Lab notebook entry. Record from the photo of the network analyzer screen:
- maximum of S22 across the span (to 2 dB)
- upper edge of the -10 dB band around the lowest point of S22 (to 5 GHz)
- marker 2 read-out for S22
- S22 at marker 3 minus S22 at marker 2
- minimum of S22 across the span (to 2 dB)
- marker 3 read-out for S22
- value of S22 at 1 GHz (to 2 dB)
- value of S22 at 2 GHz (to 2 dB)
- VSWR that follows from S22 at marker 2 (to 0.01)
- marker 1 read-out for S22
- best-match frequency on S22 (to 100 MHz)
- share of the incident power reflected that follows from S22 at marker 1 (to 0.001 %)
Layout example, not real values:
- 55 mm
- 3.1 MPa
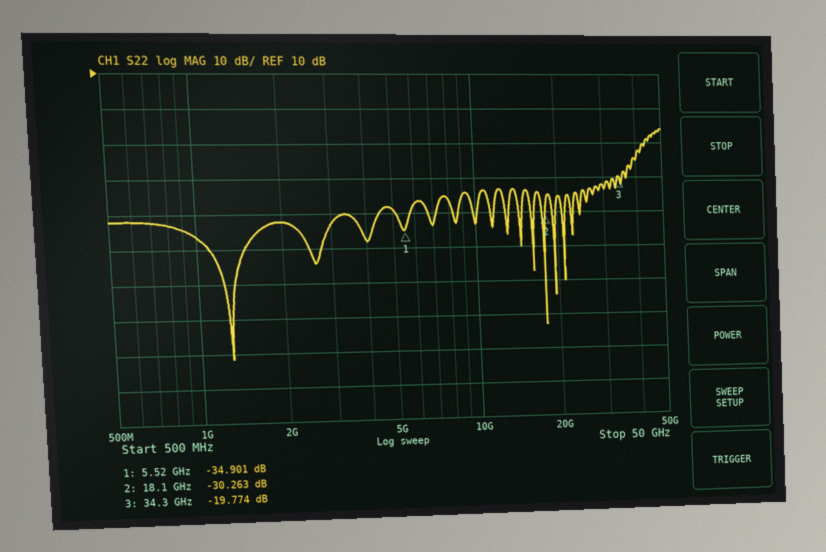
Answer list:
- -6 dB
- 45 GHz
- -30.263 dB
- 10.489 dB
- -72 dB
- -19.774 dB
- -36 dB
- -32 dB
- 1.06
- -34.901 dB
- 1.3 GHz
- 0.032 %
